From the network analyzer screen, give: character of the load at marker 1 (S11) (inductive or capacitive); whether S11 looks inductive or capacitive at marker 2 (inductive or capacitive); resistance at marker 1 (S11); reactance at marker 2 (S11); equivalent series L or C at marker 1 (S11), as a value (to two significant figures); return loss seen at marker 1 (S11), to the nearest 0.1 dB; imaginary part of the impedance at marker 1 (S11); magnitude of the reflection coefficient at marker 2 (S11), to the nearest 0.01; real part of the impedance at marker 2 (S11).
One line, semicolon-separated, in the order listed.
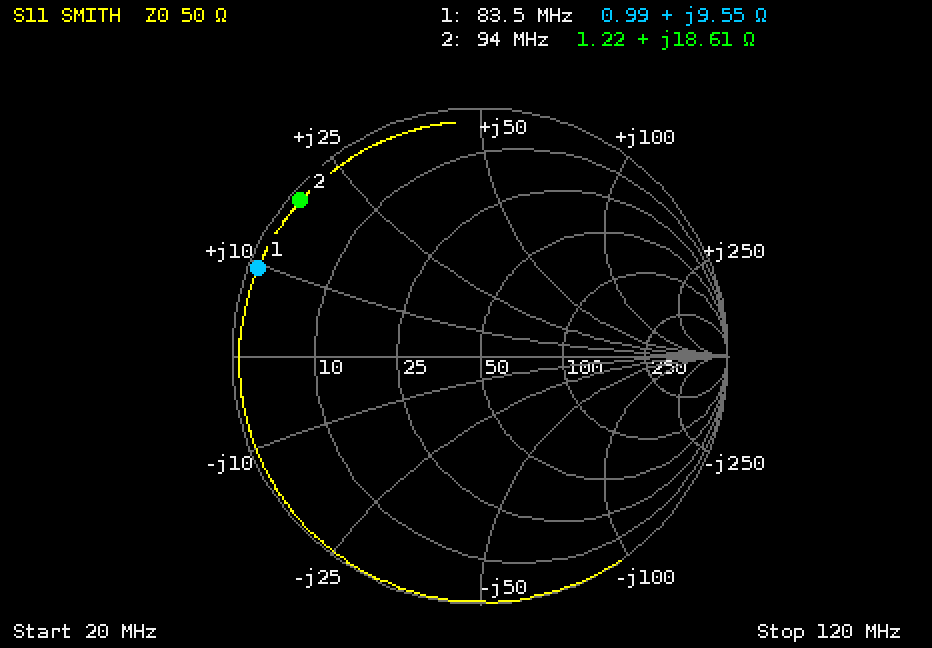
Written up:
inductive; inductive; 0.99 Ω; +18.61 Ω; 18 nH; 0.3 dB; +9.55 Ω; 0.96; 1.22 Ω
